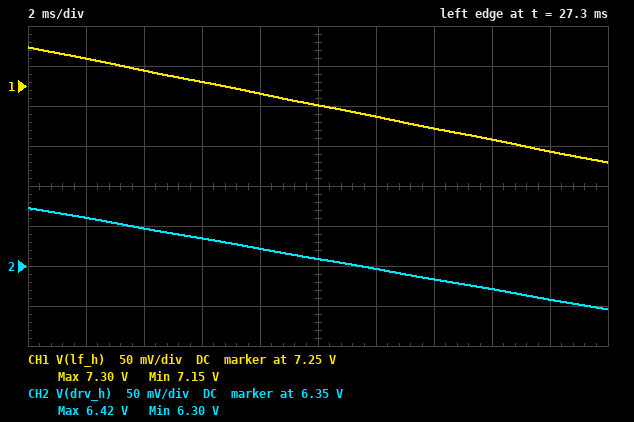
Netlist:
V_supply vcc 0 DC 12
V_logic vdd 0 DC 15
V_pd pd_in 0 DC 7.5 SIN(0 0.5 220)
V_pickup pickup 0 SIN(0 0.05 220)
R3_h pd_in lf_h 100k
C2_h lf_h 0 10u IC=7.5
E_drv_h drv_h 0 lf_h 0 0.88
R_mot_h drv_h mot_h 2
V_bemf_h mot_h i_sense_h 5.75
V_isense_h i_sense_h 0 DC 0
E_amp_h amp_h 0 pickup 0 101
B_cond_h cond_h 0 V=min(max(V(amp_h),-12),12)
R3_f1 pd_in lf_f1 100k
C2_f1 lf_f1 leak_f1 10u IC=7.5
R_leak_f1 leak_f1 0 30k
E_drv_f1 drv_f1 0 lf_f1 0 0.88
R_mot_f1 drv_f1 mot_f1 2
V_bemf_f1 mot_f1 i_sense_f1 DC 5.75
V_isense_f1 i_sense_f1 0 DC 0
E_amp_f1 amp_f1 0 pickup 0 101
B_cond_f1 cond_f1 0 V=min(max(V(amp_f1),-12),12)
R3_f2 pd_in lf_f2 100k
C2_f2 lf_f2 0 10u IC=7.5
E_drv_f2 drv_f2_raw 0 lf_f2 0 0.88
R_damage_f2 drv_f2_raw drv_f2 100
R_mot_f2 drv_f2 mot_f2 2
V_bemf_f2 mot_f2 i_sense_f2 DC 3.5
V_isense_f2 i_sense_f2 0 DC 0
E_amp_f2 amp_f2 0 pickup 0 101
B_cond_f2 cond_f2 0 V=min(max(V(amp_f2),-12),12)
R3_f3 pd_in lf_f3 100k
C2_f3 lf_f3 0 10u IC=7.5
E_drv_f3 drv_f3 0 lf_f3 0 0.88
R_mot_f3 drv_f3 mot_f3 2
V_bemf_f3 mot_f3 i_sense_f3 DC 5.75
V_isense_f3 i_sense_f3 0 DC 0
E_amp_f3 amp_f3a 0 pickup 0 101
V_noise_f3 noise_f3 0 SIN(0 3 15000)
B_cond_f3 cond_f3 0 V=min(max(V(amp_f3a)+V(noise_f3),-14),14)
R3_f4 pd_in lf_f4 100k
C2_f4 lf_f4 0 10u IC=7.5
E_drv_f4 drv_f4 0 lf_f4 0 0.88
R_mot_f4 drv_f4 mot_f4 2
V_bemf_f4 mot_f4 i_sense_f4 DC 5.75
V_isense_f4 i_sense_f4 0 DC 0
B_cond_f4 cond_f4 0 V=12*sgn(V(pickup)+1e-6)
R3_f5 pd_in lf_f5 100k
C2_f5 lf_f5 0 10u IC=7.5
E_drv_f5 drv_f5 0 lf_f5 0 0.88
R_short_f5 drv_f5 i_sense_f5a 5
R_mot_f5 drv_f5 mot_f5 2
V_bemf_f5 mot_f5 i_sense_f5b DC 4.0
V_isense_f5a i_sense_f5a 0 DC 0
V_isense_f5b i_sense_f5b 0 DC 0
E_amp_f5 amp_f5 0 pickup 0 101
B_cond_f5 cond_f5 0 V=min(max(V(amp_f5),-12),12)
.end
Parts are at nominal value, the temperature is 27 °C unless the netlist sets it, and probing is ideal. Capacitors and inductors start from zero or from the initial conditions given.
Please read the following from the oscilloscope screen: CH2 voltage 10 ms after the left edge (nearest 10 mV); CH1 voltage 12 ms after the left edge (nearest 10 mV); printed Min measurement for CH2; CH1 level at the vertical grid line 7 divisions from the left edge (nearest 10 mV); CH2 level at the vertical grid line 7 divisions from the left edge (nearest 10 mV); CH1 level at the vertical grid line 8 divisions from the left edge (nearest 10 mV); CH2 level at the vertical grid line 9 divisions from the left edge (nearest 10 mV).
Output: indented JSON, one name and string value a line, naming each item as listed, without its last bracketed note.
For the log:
{
  "CH2 voltage 10 ms after the left edge": "6.36 V",
  "CH1 voltage 12 ms after the left edge": "7.21 V",
  "printed Min measurement for CH2": "6.30 V",
  "CH1 level at the vertical grid line 7 divisions from the left edge": "7.20 V",
  "CH2 level at the vertical grid line 7 divisions from the left edge": "6.33 V",
  "CH1 level at the vertical grid line 8 divisions from the left edge": "7.18 V",
  "CH2 level at the vertical grid line 9 divisions from the left edge": "6.31 V"
}
